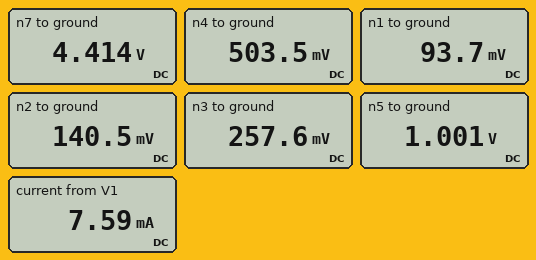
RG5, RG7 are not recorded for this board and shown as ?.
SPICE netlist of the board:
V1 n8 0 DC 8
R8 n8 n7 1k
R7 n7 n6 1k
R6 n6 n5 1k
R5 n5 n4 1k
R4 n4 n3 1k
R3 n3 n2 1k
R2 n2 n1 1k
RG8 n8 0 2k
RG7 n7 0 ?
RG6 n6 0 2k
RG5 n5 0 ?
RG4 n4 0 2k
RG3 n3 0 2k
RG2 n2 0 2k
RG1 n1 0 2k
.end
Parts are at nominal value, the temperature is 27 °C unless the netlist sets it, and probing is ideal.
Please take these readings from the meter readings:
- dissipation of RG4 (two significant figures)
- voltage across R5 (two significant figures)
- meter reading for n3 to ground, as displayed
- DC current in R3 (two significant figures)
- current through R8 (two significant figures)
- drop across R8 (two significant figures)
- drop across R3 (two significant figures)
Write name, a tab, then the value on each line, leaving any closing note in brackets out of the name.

dissipation of RG4	130 µW
voltage across R5	500 mV
meter reading for n3 to ground, as displayed	257.6 mV
DC current in R3	120 µA
current through R8	3.6 mA
drop across R8	3.6 V
drop across R3	120 mV
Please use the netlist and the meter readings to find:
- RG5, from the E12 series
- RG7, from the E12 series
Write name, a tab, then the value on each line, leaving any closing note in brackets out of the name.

RG5, from the E12 series	1.5 kΩ
RG7, from the E12 series	3.3 kΩ
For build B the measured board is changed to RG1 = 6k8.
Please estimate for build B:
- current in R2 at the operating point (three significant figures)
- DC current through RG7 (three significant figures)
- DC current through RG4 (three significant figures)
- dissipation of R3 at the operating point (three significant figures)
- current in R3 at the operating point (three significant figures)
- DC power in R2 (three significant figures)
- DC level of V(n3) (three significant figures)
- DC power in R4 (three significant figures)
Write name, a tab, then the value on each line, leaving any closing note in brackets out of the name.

current in R2 at the operating point	21.3 µA
DC current through RG7	1.34 mA
DC current through RG4	255 µA
dissipation of R3 at the operating point	10.9 µW
current in R3 at the operating point	104 µA
DC power in R2	453 nW
DC level of V(n3)	270 mV
DC power in R4	57.3 µW
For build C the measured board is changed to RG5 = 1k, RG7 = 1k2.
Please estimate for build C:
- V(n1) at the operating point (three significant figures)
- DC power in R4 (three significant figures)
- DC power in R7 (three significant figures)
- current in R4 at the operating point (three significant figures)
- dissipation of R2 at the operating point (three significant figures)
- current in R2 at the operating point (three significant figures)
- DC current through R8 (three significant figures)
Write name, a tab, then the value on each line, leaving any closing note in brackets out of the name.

V(n1) at the operating point	60.6 mV
DC power in R4	25.3 µW
DC power in R7	3.16 mW
current in R4 at the operating point	159 µA
dissipation of R2 at the operating point	917 nW
current in R2 at the operating point	30.3 µA
DC current through R8	4.61 mA
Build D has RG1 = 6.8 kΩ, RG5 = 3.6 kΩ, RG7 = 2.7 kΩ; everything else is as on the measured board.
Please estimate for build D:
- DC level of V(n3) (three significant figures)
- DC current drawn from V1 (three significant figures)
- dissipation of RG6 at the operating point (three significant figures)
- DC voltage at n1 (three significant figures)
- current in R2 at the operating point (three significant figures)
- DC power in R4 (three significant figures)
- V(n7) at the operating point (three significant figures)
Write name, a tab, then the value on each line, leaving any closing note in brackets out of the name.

DC level of V(n3)	339 mV
DC current drawn from V1	7.68 mA
dissipation of RG6 at the operating point	2.49 mW
DC voltage at n1	182 mV
current in R2 at the operating point	26.7 µA
DC power in R4	90.3 µW
V(n7) at the operating point	4.32 V
